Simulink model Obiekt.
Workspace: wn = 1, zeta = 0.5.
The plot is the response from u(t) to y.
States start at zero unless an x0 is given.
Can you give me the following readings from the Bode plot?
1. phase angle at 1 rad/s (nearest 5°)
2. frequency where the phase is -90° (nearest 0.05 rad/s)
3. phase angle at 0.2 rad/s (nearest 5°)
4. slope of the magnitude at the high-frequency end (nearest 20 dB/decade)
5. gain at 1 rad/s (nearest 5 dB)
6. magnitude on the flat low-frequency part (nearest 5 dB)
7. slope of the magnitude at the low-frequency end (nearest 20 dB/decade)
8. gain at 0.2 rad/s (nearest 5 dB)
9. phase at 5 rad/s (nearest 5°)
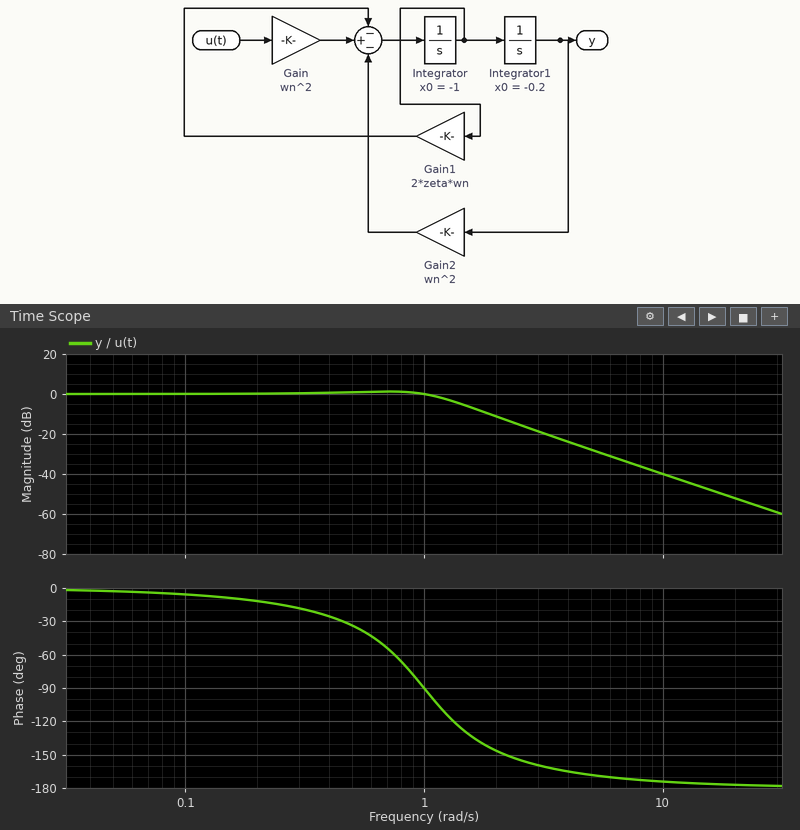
-90°
1.00 rad/s
-10°
-40 dB/decade
0 dB
0 dB
0 dB/decade
0 dB
-170°
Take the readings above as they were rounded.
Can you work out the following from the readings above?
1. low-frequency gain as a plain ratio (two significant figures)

1.0
